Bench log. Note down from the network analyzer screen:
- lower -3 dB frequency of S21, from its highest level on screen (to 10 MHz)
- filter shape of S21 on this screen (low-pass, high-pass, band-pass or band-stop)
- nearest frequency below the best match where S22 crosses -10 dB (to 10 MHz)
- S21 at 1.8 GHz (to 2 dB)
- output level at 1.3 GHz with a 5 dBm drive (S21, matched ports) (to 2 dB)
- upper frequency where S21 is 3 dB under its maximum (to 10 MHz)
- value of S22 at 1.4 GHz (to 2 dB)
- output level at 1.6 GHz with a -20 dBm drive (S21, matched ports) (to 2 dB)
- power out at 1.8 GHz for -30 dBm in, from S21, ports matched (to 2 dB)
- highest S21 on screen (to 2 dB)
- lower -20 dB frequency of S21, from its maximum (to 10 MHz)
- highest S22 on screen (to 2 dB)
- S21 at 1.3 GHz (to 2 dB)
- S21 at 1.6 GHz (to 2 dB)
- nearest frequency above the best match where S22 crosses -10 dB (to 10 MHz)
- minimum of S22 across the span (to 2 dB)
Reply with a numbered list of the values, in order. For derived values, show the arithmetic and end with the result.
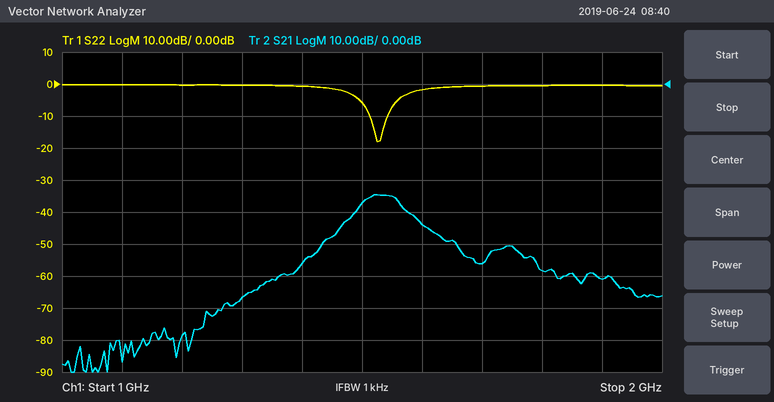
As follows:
1. 1.50 GHz
2. band-pass
3. 1.51 GHz
4. -58 dB
5. 5 dBm + (-66 dB) = -62 dBm
6. 1.56 GHz
7. 0 dB
8. -20 dBm + (-44 dB) = -64 dBm
9. -30 dBm + (-58 dB) = -88 dBm
10. -34 dB
11. 1.41 GHz
12. 0 dB
13. -66 dB
14. -44 dB
15. 1.54 GHz
16. -18 dB
